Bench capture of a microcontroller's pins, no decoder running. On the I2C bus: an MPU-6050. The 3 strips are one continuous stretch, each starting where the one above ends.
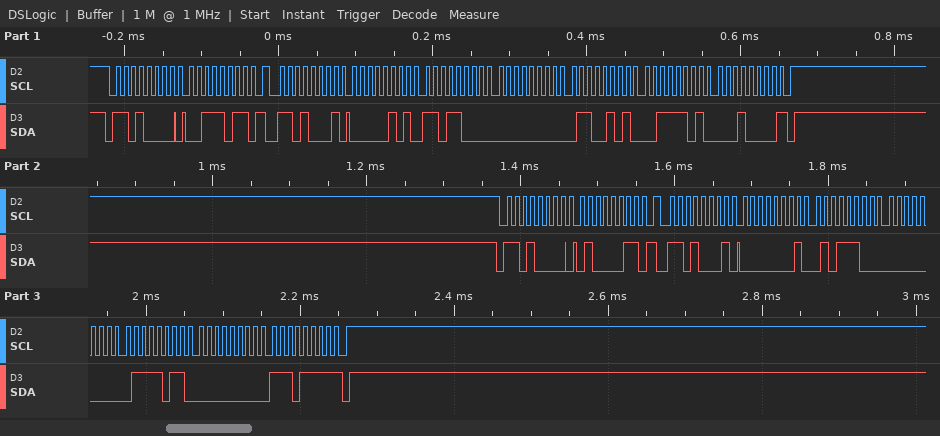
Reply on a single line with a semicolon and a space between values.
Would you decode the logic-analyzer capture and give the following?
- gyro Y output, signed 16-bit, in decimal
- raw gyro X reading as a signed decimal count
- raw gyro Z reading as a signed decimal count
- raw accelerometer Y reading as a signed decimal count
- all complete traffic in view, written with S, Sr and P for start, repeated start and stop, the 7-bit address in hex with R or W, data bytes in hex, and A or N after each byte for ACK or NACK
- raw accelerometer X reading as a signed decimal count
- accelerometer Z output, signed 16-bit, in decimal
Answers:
123; 348; 239; 101; S 68W A 3B A Sr 68R A 05 A D8 A 00 A 65 A 3D A 10 N P S 68W A 43 A Sr 68R A 01 A 5C A 00 A 7B A 00 A EF N P; 1496; 15632
